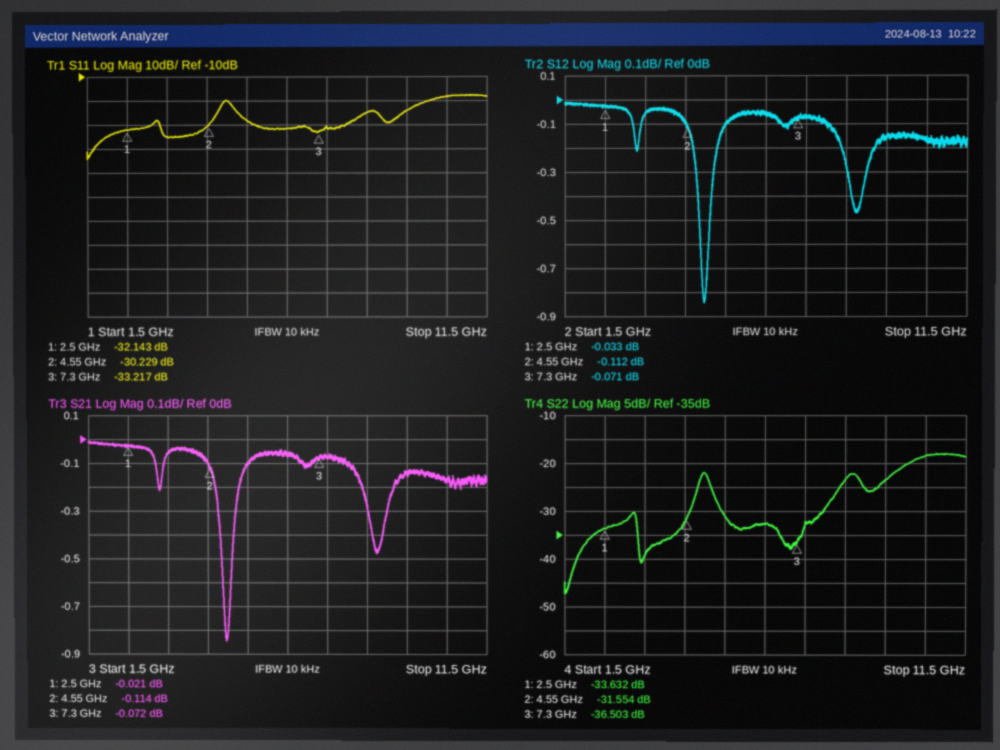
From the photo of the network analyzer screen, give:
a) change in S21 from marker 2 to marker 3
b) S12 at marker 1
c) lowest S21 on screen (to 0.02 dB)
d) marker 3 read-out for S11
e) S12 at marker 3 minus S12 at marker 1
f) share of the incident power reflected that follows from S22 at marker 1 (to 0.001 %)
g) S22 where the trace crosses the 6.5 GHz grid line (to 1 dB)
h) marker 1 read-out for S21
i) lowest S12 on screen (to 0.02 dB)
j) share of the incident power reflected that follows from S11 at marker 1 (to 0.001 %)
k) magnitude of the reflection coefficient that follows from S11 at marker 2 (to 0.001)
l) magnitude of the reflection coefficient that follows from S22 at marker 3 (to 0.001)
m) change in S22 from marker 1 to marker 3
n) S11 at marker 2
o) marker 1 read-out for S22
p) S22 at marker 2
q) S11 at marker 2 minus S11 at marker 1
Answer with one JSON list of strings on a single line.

["0.042 dB", "-0.033 dB", "-0.84 dB", "-33.217 dB", "-0.038 dB", "0.043 %", "-33 dB", "-0.021 dB", "-0.84 dB", "0.061 %", "0.031", "0.015", "-2.871 dB", "-30.229 dB", "-33.632 dB", "-31.554 dB", "1.914 dB"]
